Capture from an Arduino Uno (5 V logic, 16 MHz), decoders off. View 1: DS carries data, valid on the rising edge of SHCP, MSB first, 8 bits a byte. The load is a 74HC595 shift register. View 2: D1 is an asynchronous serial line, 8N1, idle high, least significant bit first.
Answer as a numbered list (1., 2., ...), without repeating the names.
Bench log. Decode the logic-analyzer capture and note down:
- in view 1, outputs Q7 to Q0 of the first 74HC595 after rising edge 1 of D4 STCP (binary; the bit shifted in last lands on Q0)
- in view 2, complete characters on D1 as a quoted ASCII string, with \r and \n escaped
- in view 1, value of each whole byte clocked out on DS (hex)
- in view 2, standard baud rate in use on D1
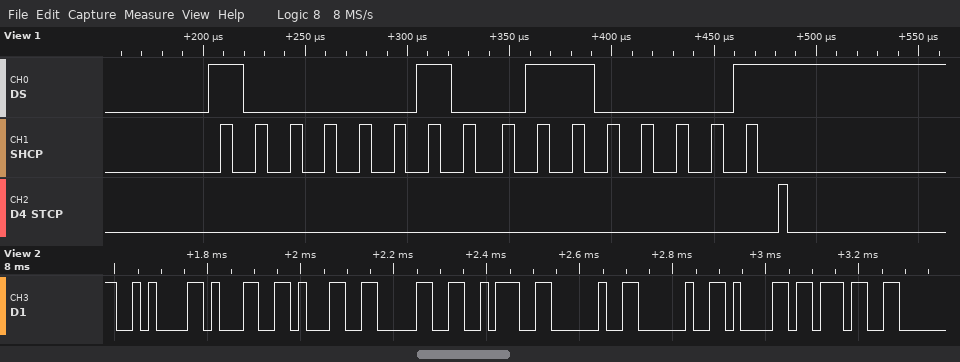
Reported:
1. 01100001
2. "\n110:  a7"
3. 0x82 0x61
4. 57600 baud
